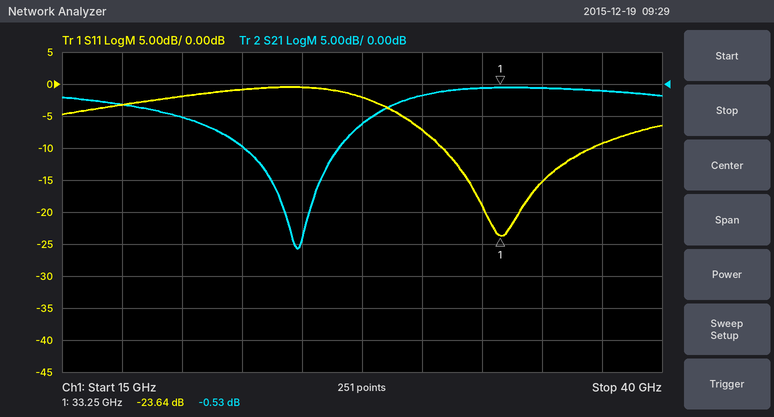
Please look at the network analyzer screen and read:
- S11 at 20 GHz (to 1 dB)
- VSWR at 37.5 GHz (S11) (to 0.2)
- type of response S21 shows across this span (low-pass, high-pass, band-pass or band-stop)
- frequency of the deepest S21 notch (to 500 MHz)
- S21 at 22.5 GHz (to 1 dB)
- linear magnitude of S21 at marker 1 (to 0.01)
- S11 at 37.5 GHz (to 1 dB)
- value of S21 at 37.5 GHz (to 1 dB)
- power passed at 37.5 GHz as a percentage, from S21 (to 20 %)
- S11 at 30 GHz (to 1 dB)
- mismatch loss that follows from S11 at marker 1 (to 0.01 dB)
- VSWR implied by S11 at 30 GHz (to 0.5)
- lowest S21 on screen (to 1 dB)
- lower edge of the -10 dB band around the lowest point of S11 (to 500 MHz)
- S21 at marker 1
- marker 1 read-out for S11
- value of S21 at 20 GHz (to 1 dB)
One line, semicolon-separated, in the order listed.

-2 dB; 2.0; band-stop; 25.0 GHz; -10 dB; 0.94; -9 dB; -1 dB; 80 %; -7 dB; 0.02 dB; 2.5; -26 dB; 31.0 GHz; -0.53 dB; -23.64 dB; -5 dB
